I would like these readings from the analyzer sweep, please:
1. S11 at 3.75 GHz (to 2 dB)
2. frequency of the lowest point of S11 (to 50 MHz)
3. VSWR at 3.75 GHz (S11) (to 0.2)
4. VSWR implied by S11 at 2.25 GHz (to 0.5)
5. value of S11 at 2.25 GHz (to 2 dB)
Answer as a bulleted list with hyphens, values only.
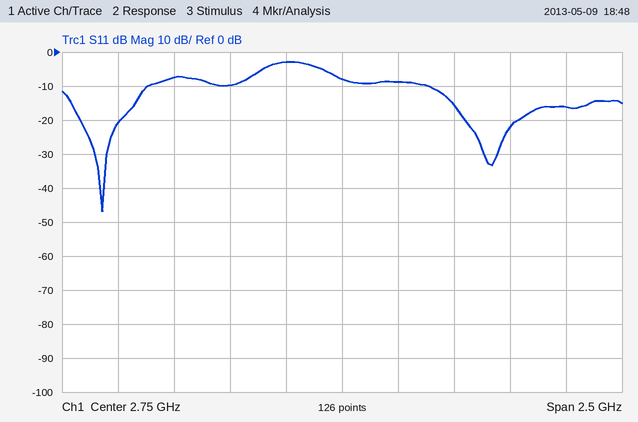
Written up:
- -16 dB
- 1.70 GHz
- 1.4
- 2.0
- -10 dB
